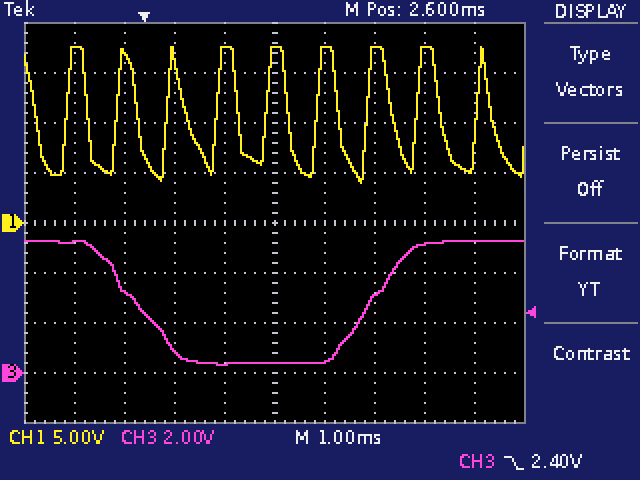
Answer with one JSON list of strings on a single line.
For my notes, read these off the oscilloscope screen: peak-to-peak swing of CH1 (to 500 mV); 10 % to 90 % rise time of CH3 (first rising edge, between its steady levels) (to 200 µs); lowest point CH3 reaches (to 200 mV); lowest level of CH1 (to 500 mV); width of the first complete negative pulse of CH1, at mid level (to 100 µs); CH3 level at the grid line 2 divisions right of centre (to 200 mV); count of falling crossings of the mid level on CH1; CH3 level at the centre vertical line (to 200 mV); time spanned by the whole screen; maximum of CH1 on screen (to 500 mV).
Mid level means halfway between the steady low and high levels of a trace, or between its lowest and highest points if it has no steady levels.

["13.5 V", "1.4 ms", "400 mV", "4.0 V", "600 µs", "3.0 V", "10", "400 mV", "10 ms", "17.5 V"]
